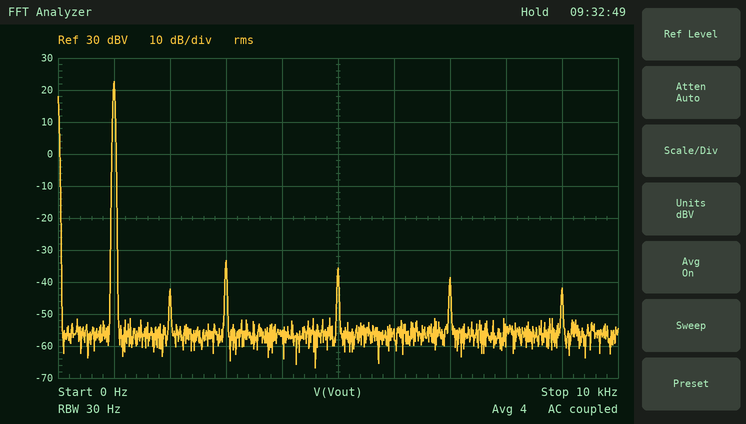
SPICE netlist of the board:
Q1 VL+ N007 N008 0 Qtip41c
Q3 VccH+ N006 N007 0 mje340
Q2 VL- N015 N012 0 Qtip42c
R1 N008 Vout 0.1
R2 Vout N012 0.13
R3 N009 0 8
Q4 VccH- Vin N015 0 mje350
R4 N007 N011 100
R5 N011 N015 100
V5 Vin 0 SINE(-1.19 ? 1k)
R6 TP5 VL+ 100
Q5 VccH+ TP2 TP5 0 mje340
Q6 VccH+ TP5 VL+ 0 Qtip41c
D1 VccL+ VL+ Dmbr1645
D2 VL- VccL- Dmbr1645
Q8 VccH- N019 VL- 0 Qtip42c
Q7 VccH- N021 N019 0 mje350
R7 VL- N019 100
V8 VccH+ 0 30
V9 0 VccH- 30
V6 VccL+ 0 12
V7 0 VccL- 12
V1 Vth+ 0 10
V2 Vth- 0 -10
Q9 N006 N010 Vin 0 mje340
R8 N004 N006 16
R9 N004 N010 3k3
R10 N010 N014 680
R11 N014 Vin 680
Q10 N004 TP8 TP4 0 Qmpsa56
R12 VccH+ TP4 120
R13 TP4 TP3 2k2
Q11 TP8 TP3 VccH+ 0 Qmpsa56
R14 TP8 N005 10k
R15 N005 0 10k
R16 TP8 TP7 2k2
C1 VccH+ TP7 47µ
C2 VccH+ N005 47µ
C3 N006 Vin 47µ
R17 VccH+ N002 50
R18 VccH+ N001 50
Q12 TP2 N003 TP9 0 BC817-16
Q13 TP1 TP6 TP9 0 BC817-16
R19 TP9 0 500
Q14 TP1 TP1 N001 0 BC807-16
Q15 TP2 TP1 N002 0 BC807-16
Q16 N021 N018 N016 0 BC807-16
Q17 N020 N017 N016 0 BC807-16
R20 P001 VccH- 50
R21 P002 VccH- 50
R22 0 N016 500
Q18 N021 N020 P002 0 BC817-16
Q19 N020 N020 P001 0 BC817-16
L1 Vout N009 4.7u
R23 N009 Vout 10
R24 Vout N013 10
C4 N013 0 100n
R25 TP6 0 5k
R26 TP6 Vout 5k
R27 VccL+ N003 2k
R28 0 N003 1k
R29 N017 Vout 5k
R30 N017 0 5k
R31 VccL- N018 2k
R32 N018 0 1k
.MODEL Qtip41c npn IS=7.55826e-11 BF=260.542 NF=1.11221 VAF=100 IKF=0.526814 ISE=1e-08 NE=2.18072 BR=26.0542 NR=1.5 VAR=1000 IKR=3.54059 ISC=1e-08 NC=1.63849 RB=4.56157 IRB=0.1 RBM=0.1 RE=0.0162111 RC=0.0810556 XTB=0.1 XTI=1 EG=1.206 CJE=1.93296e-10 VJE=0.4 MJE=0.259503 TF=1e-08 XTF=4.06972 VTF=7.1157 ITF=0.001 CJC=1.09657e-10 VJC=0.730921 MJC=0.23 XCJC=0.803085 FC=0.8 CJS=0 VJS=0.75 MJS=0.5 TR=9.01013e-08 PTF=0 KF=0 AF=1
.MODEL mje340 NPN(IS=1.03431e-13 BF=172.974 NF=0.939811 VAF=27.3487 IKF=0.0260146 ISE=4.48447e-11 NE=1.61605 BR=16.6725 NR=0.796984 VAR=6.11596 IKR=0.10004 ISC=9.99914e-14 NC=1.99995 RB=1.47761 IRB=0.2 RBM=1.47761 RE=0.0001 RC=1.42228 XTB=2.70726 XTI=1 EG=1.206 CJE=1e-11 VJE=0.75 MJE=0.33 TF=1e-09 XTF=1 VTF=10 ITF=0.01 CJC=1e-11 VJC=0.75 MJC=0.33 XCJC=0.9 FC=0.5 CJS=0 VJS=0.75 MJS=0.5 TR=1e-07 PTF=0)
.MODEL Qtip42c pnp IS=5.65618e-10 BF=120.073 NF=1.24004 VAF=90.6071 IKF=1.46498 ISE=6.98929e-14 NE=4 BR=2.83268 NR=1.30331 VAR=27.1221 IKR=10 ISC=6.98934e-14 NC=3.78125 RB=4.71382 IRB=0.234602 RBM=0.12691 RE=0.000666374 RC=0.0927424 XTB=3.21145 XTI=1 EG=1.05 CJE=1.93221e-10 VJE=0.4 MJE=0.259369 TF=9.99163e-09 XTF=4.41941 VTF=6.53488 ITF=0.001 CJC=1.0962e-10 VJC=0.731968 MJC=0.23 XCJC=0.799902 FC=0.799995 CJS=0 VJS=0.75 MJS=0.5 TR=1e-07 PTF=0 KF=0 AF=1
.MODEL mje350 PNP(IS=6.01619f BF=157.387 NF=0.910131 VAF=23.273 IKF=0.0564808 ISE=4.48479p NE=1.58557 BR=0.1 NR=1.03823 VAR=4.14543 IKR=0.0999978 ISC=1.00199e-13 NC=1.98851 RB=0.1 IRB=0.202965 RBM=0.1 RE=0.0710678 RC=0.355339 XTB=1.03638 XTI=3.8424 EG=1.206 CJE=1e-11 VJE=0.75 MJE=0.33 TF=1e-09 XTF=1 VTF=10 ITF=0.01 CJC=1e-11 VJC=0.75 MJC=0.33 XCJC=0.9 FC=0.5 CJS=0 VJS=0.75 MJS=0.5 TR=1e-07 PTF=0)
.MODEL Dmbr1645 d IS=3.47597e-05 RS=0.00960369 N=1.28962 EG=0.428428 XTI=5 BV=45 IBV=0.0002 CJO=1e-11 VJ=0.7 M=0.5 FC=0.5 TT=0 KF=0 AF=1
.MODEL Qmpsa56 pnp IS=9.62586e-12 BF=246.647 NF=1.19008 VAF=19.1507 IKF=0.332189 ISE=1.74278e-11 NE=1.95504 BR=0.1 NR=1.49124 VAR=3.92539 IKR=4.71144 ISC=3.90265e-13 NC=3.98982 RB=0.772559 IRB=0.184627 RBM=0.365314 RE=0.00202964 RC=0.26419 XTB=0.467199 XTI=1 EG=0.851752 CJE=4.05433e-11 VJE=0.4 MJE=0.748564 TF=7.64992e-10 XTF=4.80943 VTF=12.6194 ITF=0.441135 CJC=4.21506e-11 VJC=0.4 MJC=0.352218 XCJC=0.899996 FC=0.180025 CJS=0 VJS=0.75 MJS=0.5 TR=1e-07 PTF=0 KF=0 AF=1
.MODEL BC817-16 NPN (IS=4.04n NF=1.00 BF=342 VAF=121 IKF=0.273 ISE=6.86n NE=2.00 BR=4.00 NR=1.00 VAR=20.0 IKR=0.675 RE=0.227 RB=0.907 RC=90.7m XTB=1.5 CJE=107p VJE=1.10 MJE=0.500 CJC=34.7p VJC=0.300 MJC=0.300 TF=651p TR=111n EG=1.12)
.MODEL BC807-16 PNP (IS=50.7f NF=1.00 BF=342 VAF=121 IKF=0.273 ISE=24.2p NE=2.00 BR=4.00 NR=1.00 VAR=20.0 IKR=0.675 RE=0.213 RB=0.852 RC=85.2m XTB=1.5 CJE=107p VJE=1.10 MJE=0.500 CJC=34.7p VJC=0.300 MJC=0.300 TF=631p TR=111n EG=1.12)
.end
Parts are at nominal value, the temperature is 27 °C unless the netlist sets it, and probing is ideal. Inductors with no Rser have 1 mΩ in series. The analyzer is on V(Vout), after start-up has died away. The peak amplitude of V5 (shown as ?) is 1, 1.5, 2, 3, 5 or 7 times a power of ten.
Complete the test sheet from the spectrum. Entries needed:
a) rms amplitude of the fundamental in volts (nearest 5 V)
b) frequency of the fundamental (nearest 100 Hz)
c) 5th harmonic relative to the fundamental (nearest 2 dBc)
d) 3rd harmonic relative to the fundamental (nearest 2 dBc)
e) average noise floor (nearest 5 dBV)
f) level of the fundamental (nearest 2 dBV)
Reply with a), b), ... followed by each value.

a) 15 V
b) 1.0 kHz
c) -58 dBc
d) -56 dBc
e) -55 dBV
f) 22 dBV
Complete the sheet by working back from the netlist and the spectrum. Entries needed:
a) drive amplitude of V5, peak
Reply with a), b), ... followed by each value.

a) 20 V
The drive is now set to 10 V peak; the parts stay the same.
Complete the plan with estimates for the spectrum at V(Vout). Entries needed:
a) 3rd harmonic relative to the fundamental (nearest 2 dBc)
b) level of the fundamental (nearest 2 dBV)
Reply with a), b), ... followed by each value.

a) -48 dBc
b) 16 dBV
